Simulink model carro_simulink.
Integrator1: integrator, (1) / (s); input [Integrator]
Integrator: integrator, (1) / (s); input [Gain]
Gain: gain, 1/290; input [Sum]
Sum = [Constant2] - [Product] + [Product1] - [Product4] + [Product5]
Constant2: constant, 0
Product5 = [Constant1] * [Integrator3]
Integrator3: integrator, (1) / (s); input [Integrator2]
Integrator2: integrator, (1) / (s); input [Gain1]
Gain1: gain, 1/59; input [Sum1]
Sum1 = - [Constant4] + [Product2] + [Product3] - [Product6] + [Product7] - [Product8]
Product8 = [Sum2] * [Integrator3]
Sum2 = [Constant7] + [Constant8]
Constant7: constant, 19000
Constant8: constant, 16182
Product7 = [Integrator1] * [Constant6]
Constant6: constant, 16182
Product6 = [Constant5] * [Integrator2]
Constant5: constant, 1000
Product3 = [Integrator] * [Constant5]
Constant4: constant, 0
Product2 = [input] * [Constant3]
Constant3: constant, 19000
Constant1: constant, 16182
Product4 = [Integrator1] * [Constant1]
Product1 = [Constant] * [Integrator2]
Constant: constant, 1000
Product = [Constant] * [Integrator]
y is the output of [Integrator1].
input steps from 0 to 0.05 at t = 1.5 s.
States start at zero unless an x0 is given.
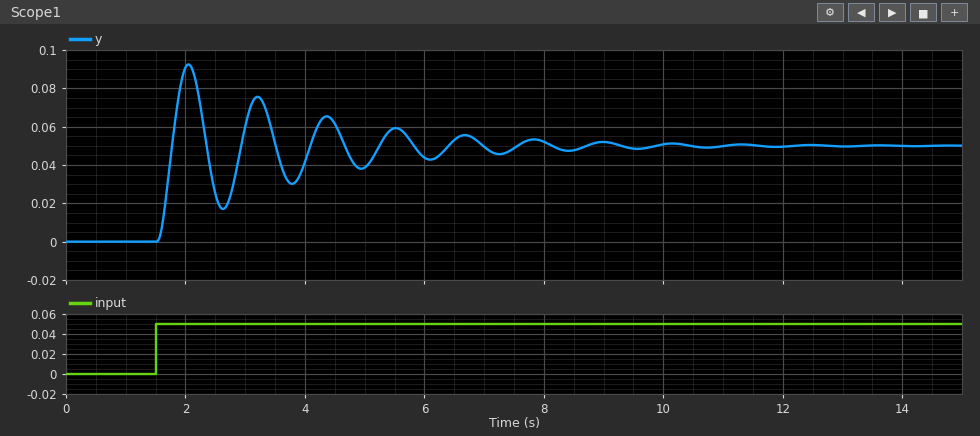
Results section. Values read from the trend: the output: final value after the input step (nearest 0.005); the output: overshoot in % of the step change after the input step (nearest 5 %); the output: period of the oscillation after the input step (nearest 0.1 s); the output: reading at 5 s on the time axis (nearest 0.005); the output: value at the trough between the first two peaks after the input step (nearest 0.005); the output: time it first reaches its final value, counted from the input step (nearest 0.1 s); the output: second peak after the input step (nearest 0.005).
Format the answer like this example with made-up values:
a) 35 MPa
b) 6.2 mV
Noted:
a) 0.050
b) 85 %
c) 1.2 s
d) 0.040
e) 0.015
f) 0.3 s
g) 0.075
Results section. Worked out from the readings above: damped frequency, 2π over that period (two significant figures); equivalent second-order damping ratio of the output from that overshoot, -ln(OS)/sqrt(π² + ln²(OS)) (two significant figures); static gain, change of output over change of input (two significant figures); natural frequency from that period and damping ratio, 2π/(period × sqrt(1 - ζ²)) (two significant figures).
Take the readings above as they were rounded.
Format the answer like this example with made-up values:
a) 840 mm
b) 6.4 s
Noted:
a) 5.2 rad/s
b) 0.052
c) 1.0
d) 5.2 rad/s
